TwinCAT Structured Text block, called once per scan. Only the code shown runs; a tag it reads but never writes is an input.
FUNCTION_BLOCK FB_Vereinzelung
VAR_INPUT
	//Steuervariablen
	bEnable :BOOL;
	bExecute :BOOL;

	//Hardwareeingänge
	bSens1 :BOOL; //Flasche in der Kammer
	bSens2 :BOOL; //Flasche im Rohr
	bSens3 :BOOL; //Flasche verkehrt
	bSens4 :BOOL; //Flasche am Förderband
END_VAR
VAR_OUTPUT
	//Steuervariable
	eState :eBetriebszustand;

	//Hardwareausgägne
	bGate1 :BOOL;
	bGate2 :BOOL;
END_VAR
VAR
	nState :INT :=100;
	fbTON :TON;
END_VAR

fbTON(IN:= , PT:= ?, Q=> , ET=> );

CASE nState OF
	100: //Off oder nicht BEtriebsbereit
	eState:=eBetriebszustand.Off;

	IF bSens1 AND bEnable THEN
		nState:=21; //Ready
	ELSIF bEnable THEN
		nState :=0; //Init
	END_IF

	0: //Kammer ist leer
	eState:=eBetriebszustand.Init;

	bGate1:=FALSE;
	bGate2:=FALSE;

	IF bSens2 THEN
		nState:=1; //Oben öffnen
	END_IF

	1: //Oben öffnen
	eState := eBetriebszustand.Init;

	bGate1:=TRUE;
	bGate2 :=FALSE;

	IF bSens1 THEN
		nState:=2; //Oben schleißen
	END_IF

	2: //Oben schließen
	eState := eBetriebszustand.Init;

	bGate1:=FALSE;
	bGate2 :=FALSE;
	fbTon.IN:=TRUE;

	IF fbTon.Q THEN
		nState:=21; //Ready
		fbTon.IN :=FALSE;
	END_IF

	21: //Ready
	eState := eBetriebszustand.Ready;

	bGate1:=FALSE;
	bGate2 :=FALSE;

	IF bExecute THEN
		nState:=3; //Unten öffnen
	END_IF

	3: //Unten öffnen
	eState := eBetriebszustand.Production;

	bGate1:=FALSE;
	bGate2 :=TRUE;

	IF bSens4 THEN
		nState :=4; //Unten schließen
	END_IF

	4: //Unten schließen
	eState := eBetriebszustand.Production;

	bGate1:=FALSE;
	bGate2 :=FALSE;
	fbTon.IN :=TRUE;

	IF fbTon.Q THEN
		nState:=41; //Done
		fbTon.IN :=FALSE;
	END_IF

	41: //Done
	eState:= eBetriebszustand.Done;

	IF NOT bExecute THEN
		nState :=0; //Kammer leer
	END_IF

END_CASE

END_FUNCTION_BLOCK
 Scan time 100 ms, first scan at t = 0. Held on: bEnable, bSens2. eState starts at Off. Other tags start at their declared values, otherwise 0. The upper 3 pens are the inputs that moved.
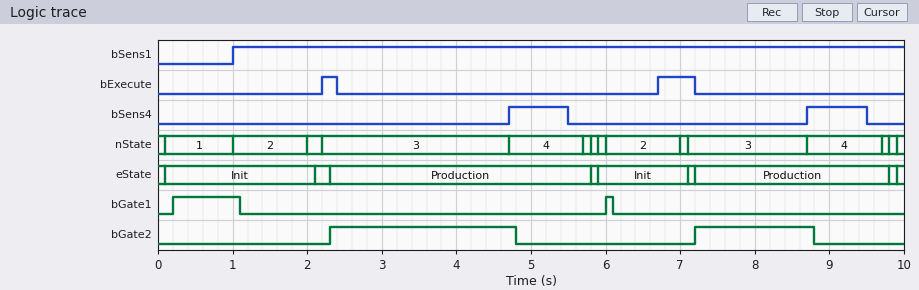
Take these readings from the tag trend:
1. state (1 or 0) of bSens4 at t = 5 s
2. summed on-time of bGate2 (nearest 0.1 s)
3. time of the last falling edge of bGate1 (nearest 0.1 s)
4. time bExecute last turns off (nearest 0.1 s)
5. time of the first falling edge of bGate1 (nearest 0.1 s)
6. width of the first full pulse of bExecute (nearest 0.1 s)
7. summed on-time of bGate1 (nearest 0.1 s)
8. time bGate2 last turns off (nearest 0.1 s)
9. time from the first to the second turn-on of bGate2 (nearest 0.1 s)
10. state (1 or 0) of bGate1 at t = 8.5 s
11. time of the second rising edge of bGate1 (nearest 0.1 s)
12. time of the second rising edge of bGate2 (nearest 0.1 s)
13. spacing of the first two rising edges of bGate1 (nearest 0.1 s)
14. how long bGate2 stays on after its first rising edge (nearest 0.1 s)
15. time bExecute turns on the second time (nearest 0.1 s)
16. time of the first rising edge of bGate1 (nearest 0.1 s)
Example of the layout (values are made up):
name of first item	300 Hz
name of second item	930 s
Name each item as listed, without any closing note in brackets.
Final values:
state (1 or 0) of bSens4 at t = 5 s	1
summed on-time of bGate2	4.1 s
time of the last falling edge of bGate1	6.1 s
time bExecute last turns off	7.2 s
time of the first falling edge of bGate1	1.1 s
width of the first full pulse of bExecute	0.2 s
summed on-time of bGate1	1.0 s
time bGate2 last turns off	8.8 s
time from the first to the second turn-on of bGate2	4.9 s
state (1 or 0) of bGate1 at t = 8.5 s	0
time of the second rising edge of bGate1	6.0 s
time of the second rising edge of bGate2	7.2 s
spacing of the first two rising edges of bGate1	5.8 s
how long bGate2 stays on after its first rising edge	2.5 s
time bExecute turns on the second time	6.7 s
time of the first rising edge of bGate1	0.2 s
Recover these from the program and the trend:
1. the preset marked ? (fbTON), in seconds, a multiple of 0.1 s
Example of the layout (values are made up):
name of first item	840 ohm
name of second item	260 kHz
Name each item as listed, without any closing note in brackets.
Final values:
the preset marked ? (fbTON), in seconds, a multiple of 0.1 s	0.8 s
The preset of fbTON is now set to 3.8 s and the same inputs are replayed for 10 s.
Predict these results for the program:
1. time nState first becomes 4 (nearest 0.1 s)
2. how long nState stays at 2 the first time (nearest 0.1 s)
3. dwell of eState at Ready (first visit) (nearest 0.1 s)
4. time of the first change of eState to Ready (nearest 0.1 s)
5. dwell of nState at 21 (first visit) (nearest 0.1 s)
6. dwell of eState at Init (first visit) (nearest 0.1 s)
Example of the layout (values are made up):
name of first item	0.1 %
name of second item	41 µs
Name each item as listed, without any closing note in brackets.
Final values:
time nState first becomes 4	8.7 s
how long nState stays at 2 the first time	4.0 s
dwell of eState at Ready (first visit)	1.7 s
time of the first change of eState to Ready	5.1 s
dwell of nState at 21 (first visit)	1.7 s
dwell of eState at Init (first visit)	5.0 s
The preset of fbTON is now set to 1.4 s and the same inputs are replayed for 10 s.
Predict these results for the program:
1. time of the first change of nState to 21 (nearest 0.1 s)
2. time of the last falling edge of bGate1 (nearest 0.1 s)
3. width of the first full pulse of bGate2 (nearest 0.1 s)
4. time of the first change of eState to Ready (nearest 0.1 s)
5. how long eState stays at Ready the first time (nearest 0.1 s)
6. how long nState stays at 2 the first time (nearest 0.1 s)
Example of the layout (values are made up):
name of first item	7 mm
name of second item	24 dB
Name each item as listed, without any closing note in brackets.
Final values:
time of the first change of nState to 21	2.6 s
time of the last falling edge of bGate1	1.1 s
width of the first full pulse of bGate2	2.0 s
time of the first change of eState to Ready	2.7 s
how long eState stays at Ready the first time	4.1 s
how long nState stays at 2 the first time	1.6 s
